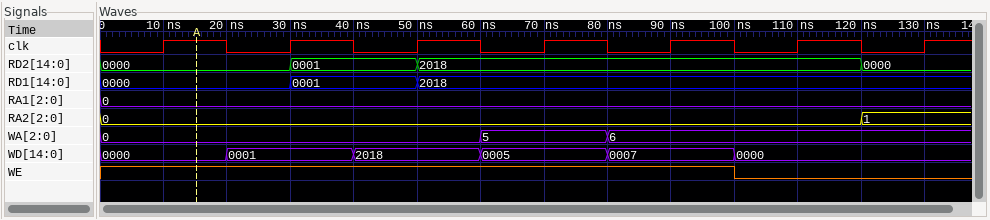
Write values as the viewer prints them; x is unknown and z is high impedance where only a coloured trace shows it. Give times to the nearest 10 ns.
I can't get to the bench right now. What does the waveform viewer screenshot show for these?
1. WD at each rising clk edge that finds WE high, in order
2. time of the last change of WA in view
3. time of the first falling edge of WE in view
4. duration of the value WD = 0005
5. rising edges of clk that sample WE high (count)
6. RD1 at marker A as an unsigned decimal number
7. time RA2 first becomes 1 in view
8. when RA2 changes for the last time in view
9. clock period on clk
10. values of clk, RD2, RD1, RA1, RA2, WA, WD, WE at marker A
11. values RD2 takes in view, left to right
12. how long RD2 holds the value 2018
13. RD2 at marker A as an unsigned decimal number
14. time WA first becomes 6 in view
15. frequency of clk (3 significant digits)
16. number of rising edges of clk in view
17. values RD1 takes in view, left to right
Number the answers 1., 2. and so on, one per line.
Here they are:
1. 0000, 0001, 2018, 0005, 0007
2. 80 ns
3. 100 ns
4. 20 ns
5. 5
6. 0
7. 120 ns
8. 120 ns
9. 20 ns
10. clk=1, RD2=0000, RD1=0000, RA1=0, RA2=0, WA=0, WD=0000, WE=1
11. 0000, 0001, 2018, 0000
12. 70 ns
13. 0
14. 80 ns
15. 50.0 MHz
16. 7
17. 0000, 0001, 2018
